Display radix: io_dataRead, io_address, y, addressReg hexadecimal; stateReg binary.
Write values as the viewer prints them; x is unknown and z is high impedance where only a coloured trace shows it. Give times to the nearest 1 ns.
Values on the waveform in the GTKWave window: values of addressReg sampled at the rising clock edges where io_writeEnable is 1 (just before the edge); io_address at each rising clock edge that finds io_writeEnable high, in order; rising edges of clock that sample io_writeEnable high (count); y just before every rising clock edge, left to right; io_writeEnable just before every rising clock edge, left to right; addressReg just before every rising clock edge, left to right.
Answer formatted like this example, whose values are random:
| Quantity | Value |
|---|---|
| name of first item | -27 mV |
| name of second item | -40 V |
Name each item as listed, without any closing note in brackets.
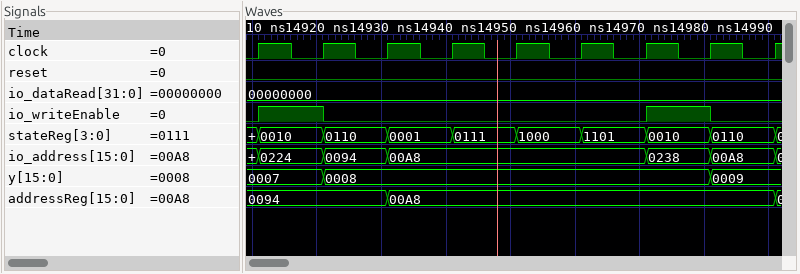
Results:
| Quantity | Value |
|---|---|
| values of addressReg sampled at the rising clock edges where io_writeEnable is 1 | 0094, 00A8 |
| io_address at each rising clock edge that finds io_writeEnable high, in order | 0224, 0238 |
| rising edges of clock that sample io_writeEnable high | 2 |
| y just before every rising clock edge, left to right | 0007, 0007, 0008, 0008, 0008, 0008, 0008, 0008, 0009 |
| io_writeEnable just before every rising clock edge, left to right | 0 1 0 0 0 0 0 1 0 |
| addressReg just before every rising clock edge, left to right | 0094, 0094, 0094, 00A8, 00A8, 00A8, 00A8, 00A8, 00A8 |
